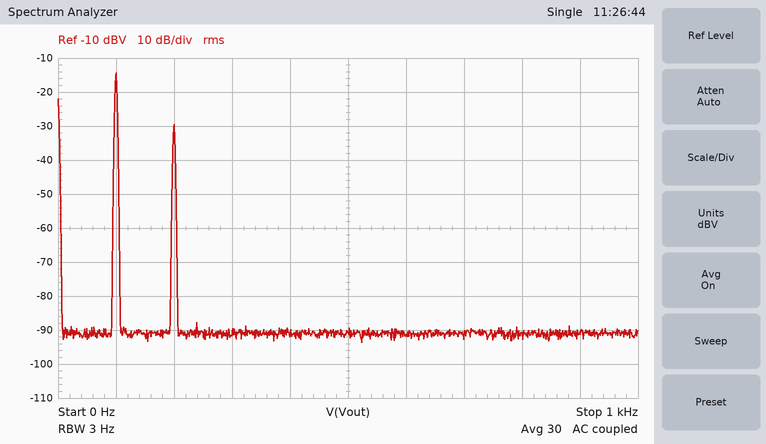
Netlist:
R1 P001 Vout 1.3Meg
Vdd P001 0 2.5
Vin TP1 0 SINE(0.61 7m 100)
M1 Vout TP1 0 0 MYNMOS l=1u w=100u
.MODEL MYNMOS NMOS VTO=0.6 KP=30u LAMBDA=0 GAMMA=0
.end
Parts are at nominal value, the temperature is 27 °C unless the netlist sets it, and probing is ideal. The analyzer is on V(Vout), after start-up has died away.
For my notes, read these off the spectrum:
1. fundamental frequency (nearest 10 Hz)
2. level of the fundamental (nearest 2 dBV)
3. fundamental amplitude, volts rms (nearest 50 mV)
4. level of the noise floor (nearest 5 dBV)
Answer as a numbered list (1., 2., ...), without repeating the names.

1. 100 Hz
2. -14 dBV
3. 200 mV
4. -90 dBV
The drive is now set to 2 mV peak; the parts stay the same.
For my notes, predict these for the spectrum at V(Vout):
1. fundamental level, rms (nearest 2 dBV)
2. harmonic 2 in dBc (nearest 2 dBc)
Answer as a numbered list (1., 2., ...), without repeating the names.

1. -26 dBV
2. -26 dBc
